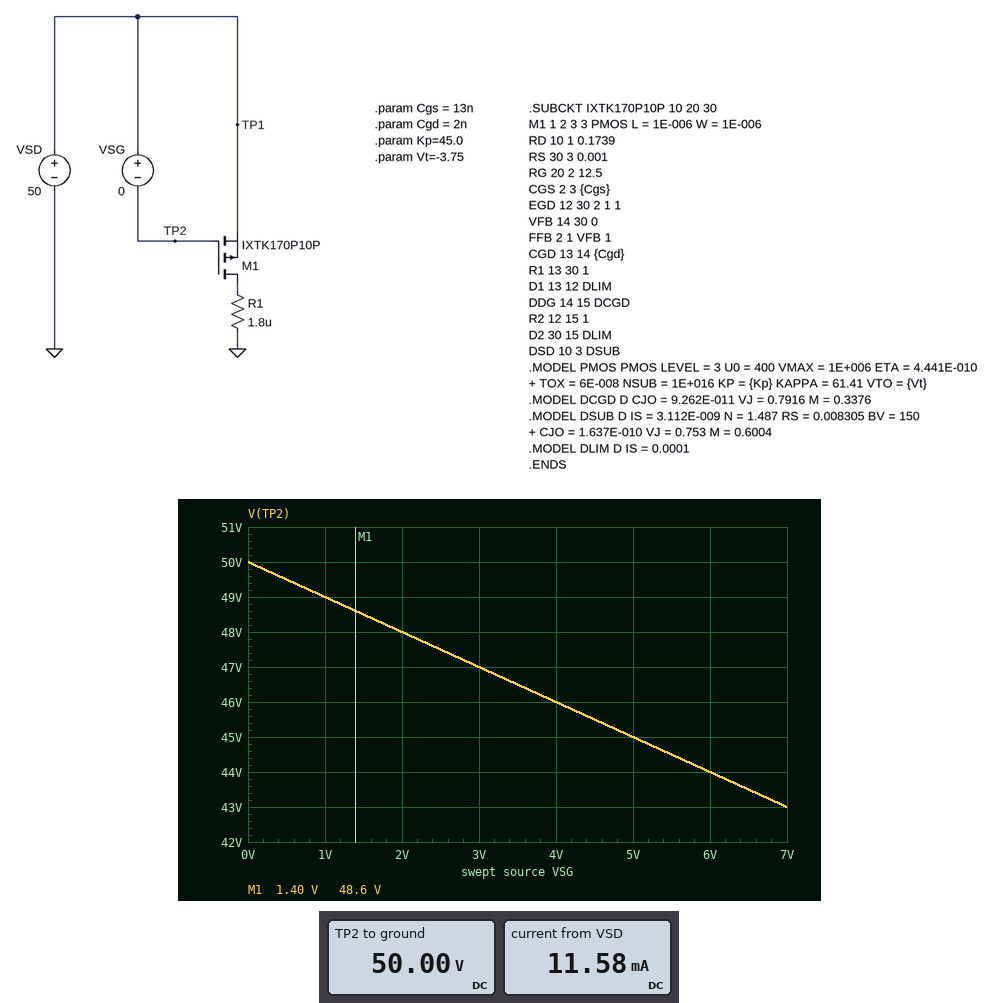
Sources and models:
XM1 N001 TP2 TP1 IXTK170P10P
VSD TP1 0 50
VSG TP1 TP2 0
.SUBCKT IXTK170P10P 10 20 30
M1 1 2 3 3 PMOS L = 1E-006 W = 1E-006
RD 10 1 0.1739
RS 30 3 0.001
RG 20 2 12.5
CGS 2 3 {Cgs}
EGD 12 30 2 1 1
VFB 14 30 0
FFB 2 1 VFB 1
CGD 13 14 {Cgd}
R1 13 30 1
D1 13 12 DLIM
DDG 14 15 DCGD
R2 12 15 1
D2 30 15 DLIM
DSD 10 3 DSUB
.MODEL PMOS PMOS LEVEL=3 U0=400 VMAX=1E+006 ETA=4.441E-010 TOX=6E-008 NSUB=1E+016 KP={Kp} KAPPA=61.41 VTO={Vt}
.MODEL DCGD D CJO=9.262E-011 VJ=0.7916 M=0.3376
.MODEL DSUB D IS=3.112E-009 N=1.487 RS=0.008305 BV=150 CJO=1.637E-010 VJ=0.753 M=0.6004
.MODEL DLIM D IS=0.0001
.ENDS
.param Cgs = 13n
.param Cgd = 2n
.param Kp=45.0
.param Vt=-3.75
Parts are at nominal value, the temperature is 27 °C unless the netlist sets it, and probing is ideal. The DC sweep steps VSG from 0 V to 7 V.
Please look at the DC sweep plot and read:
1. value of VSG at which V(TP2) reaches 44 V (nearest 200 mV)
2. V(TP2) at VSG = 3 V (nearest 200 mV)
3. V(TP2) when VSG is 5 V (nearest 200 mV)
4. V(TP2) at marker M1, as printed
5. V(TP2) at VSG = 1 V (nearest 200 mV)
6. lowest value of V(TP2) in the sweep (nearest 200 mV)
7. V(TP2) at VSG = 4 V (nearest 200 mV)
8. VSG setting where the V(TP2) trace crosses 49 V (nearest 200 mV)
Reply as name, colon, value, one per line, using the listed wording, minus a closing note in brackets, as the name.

value of VSG at which V(TP2) reaches 44 V: 6.0 V
V(TP2) at VSG = 3 V: 47.0 V
V(TP2) when VSG is 5 V: 45.0 V
V(TP2) at marker M1, as printed: 48.6 V
V(TP2) at VSG = 1 V: 49.0 V
lowest value of V(TP2) in the sweep: 43.0 V
V(TP2) at VSG = 4 V: 46.0 V
VSG setting where the V(TP2) trace crosses 49 V: 1.0 V
